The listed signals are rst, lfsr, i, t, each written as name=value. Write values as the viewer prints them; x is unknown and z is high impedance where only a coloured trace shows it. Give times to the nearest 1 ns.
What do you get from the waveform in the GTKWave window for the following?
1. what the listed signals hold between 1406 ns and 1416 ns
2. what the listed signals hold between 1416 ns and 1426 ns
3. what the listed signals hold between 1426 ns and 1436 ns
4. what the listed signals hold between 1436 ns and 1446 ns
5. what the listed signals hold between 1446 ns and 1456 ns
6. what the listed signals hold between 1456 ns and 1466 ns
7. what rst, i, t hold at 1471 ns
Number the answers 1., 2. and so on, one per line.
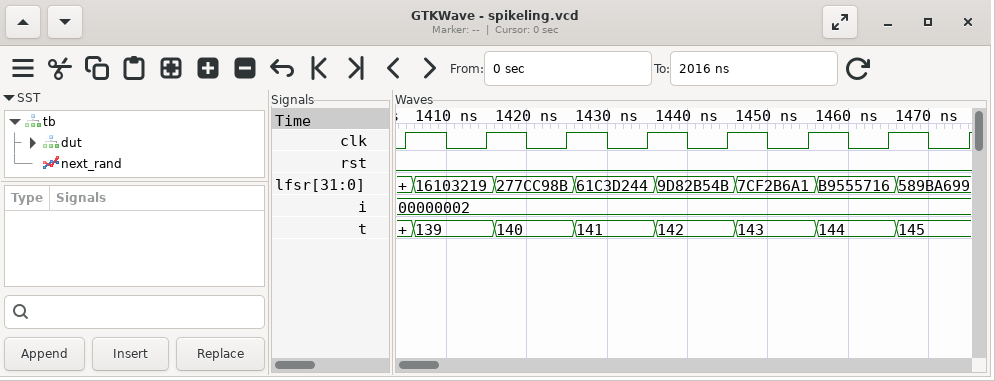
1. rst=0, lfsr=16103219, i=00000002, t=139
2. rst=0, lfsr=277CC98B, i=00000002, t=140
3. rst=0, lfsr=61C3D244, i=00000002, t=141
4. rst=0, lfsr=9D82B54B, i=00000002, t=142
5. rst=0, lfsr=7CF2B6A1, i=00000002, t=143
6. rst=0, lfsr=B9555716, i=00000002, t=144
7. rst=0, i=00000002, t=145
